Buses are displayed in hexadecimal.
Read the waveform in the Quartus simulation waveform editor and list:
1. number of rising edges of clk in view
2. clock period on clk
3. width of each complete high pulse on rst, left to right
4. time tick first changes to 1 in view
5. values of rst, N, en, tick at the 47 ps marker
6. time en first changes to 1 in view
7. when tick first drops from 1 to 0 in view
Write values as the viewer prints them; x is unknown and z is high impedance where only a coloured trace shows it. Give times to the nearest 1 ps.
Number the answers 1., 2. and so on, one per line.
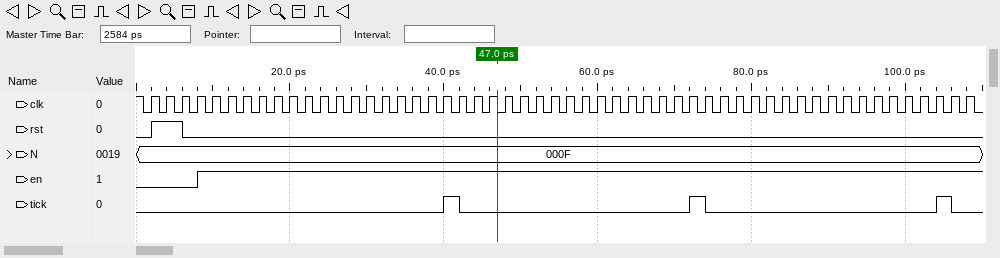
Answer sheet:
1. 54
2. 2 ps
3. 4 ps
4. 40 ps
5. rst=0, N=000F, en=1, tick=0
6. 8 ps
7. 42 ps
